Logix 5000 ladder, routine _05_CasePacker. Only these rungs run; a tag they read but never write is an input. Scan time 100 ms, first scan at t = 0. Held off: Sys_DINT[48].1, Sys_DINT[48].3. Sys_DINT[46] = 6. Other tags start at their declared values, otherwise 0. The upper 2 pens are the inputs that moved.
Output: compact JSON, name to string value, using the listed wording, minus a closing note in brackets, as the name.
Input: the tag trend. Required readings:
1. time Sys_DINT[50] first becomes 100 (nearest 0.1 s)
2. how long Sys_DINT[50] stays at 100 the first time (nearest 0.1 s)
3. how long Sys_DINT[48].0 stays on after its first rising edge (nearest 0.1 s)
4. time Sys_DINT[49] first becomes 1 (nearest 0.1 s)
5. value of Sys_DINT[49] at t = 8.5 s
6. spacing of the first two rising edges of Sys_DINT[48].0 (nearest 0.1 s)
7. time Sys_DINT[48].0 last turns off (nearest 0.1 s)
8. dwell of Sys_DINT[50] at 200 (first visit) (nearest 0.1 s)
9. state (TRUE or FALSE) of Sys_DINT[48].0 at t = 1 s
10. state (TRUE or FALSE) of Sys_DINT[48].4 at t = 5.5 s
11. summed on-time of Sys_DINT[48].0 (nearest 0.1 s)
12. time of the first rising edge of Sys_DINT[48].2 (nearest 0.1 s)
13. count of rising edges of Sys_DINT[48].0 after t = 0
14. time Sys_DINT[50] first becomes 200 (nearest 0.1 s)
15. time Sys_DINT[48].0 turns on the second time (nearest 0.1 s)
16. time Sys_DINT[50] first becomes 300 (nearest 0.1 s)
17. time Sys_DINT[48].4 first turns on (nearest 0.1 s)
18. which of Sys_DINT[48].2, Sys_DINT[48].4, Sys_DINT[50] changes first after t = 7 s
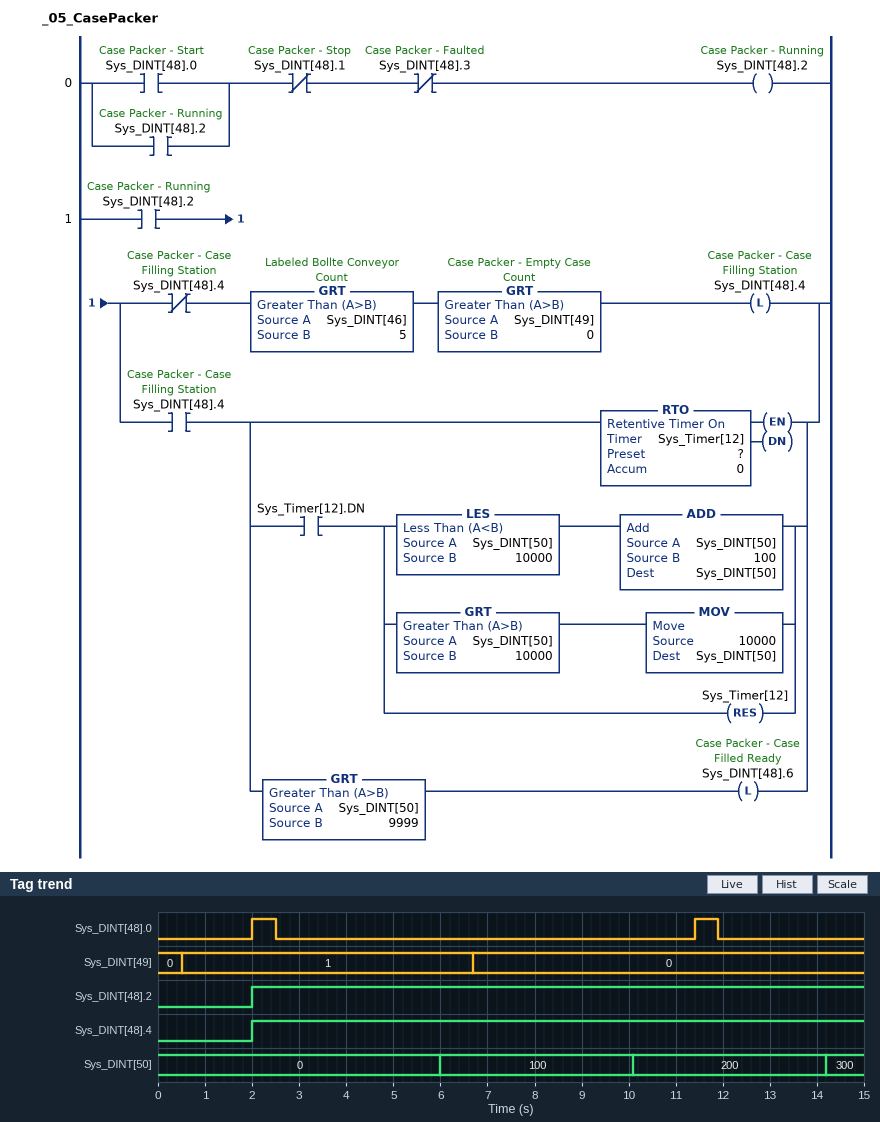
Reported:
{"time Sys_DINT[50] first becomes 100": "6.0 s", "how long Sys_DINT[50] stays at 100 the first time": "4.1 s", "how long Sys_DINT[48].0 stays on after its first rising edge": "0.5 s", "time Sys_DINT[49] first becomes 1": "0.5 s", "value of Sys_DINT[49] at t = 8.5 s": "0", "spacing of the first two rising edges of Sys_DINT[48].0": "9.4 s", "time Sys_DINT[48].0 last turns off": "11.9 s", "dwell of Sys_DINT[50] at 200 (first visit)": "4.1 s", "state (TRUE or FALSE) of Sys_DINT[48].0 at t = 1 s": "FALSE", "state (TRUE or FALSE) of Sys_DINT[48].4 at t = 5.5 s": "TRUE", "summed on-time of Sys_DINT[48].0": "1.0 s", "time of the first rising edge of Sys_DINT[48].2": "2.0 s", "count of rising edges of Sys_DINT[48].0 after t = 0": "2", "time Sys_DINT[50] first becomes 200": "10.1 s", "time Sys_DINT[48].0 turns on the second time": "11.4 s", "time Sys_DINT[50] first becomes 300": "14.2 s", "time Sys_DINT[48].4 first turns on": "2.0 s", "which of Sys_DINT[48].2, Sys_DINT[48].4, Sys_DINT[50] changes first after t = 7 s": "Sys_DINT[50]"}
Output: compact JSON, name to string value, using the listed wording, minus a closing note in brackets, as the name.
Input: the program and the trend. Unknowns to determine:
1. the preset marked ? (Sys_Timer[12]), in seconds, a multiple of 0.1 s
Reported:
{"the preset marked ? (Sys_Timer[12]), in seconds, a multiple of 0.1 s": "4.0 s"}
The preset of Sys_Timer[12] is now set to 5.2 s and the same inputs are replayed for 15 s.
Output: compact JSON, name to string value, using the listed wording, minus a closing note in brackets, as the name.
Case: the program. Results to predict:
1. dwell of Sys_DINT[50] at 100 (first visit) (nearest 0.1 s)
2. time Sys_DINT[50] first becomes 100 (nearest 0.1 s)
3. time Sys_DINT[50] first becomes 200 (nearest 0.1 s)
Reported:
{"dwell of Sys_DINT[50] at 100 (first visit)": "5.3 s", "time Sys_DINT[50] first becomes 100": "7.2 s", "time Sys_DINT[50] first becomes 200": "12.5 s"}
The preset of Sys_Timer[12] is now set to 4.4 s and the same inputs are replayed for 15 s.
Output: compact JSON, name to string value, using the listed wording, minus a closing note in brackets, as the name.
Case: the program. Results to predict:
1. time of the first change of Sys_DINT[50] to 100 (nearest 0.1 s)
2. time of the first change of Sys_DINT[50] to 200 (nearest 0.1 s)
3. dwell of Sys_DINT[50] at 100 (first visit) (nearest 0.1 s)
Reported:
{"time of the first change of Sys_DINT[50] to 100": "6.4 s", "time of the first change of Sys_DINT[50] to 200": "10.9 s", "dwell of Sys_DINT[50] at 100 (first visit)": "4.5 s"}
